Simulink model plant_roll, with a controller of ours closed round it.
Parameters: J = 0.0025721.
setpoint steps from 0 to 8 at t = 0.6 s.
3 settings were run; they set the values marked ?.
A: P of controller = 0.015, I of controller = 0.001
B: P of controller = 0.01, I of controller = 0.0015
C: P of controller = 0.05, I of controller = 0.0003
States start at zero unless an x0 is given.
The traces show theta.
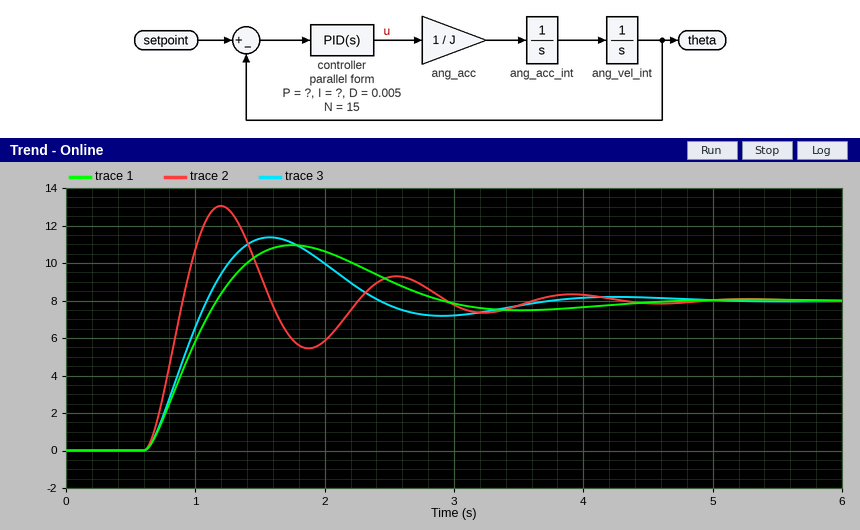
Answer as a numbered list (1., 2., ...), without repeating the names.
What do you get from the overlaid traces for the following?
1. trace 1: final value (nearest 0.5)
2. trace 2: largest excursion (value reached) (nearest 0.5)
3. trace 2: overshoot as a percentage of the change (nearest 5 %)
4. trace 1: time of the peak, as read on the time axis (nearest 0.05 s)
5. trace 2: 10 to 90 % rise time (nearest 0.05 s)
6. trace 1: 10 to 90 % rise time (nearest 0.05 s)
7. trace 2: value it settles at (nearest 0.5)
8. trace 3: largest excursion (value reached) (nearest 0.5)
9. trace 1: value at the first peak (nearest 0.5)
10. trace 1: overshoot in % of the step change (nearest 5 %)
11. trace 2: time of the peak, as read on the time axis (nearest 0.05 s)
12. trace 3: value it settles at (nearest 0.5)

1. 8.0
2. 13.0
3. 65 %
4. 1.75 s
5. 0.20 s
6. 0.40 s
7. 8.0
8. 11.5
9. 11.0
10. 35 %
11. 1.20 s
12. 8.0
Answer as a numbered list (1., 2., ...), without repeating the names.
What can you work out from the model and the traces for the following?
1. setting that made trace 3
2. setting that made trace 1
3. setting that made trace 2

1. A
2. B
3. C
